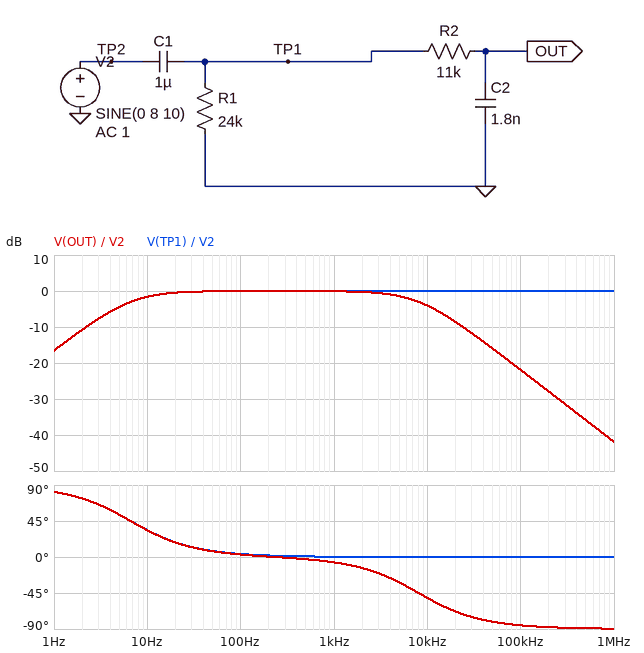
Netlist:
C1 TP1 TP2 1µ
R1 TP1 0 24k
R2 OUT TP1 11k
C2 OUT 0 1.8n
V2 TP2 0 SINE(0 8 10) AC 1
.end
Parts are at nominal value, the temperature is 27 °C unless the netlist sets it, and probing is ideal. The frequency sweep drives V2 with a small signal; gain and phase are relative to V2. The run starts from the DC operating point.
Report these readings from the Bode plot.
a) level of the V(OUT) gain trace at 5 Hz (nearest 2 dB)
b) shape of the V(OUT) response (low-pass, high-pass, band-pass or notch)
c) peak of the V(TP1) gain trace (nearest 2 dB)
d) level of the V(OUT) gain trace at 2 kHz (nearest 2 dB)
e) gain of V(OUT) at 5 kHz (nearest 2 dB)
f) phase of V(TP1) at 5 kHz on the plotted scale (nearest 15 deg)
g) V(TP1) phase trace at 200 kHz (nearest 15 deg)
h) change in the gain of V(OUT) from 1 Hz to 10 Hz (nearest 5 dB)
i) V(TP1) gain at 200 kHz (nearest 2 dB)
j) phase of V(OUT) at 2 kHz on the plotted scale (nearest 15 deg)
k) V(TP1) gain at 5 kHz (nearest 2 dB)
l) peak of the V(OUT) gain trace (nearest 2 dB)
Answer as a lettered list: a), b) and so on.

a) -4 dB
b) band-pass
c) 0 dB
d) 0 dB
e) -2 dB
f) 0 deg
g) 0 deg
h) 15 dB
i) 0 dB
j) -15 deg
k) 0 dB
l) 0 dB
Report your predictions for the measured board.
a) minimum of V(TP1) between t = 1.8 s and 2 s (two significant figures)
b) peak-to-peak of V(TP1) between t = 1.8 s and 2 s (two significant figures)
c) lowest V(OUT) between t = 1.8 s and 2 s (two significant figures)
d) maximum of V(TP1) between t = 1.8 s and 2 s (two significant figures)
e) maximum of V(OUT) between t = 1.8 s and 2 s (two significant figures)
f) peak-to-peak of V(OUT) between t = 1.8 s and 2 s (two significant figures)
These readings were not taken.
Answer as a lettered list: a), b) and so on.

a) -6.7 V
b) 13 V
c) -6.7 V
d) 6.7 V
e) 6.7 V
f) 13 V
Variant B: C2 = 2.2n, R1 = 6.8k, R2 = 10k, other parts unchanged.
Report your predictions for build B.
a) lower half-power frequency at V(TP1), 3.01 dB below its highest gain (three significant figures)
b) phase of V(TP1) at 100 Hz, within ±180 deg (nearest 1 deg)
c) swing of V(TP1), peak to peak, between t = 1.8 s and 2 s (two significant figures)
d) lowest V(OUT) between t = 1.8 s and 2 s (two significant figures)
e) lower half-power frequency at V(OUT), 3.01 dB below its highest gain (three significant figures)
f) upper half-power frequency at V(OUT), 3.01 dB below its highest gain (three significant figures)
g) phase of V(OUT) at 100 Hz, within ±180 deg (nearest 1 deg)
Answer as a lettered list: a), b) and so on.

a) 23.5 Hz
b) 13 deg
c) 6.3 V
d) -3.1 V
e) 23.2 Hz
f) 7.30 kHz
g) 12 deg
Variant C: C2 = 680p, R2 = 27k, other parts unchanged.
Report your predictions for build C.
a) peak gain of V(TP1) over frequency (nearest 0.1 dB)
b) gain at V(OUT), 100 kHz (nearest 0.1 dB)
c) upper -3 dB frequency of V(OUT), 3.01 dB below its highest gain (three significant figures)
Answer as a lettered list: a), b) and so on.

a) 0 dB
b) -21.3 dB
c) 8.69 kHz
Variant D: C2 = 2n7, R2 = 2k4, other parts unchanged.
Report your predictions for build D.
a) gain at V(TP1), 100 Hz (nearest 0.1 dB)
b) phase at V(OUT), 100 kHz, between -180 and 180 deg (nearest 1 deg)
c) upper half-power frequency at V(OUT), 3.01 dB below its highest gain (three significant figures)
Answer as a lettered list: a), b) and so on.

a) 0 dB
b) -76 deg
c) 24.6 kHz
